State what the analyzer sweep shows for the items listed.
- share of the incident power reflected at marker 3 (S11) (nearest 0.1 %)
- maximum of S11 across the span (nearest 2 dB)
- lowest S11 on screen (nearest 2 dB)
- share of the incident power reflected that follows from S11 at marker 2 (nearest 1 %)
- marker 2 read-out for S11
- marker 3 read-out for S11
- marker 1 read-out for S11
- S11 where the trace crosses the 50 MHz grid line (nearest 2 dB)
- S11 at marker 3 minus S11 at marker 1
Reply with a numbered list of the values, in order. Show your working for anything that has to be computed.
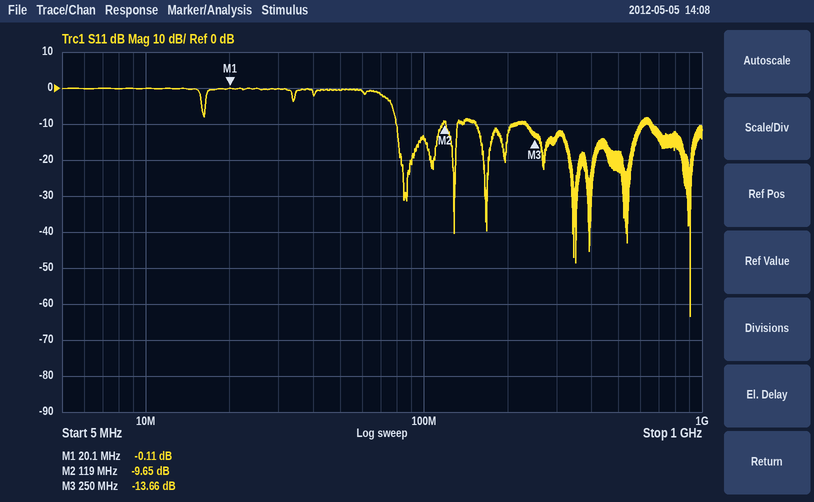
1. 10^(-13.66/10) ≈ 4.3 %
2. 0 dB
3. -64 dB
4. 10^(-9.65/10) ≈ 11 %
5. -9.65 dB
6. -13.66 dB
7. -0.11 dB
8. 0 dB
9. -13.66 − (-0.11) = -13.55 dB
